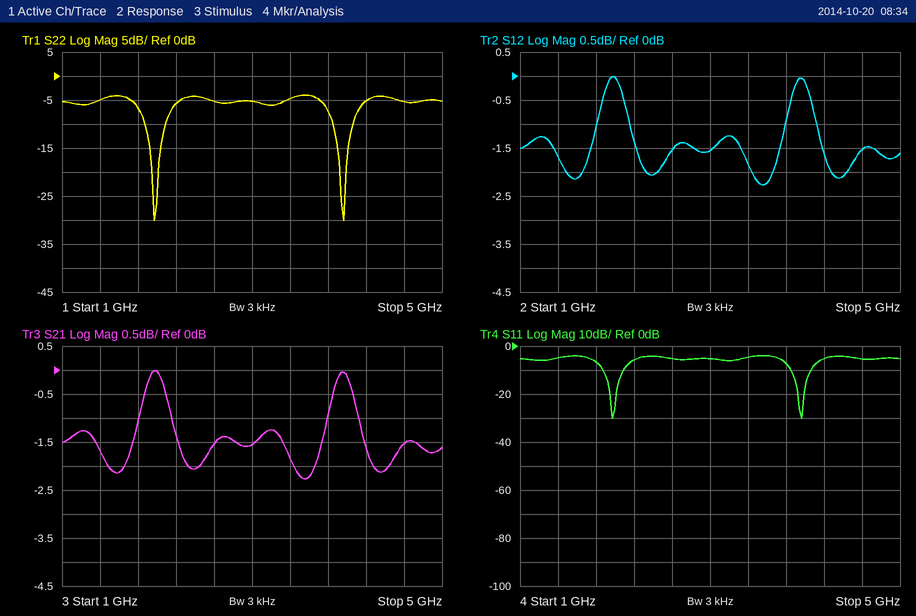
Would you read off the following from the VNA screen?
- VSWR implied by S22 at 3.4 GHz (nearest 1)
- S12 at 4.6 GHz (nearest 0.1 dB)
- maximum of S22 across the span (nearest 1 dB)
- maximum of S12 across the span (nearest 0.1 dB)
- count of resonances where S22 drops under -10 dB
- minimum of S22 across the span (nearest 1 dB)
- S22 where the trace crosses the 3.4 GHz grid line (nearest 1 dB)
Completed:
4
-1.5 dB
-4 dB
0.0 dB
2
-30 dB
-5 dB
